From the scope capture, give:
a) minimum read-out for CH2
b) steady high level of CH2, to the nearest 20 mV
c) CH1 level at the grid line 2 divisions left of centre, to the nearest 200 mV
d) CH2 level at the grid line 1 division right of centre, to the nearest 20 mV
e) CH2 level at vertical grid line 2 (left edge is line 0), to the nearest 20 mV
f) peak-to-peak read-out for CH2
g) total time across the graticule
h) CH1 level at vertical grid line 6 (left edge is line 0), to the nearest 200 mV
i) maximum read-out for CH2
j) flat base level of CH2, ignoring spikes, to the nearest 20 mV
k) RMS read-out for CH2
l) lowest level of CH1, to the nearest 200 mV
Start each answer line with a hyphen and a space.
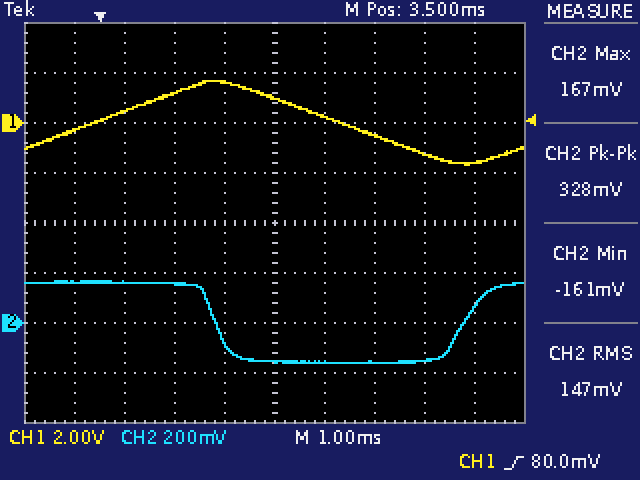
- -161 mV
- 160 mV
- 1.2 V
- -160 mV
- 160 mV
- 328 mV
- 10 ms
- 200 mV
- 167 mV
- -160 mV
- 147 mV
- -1.6 V
